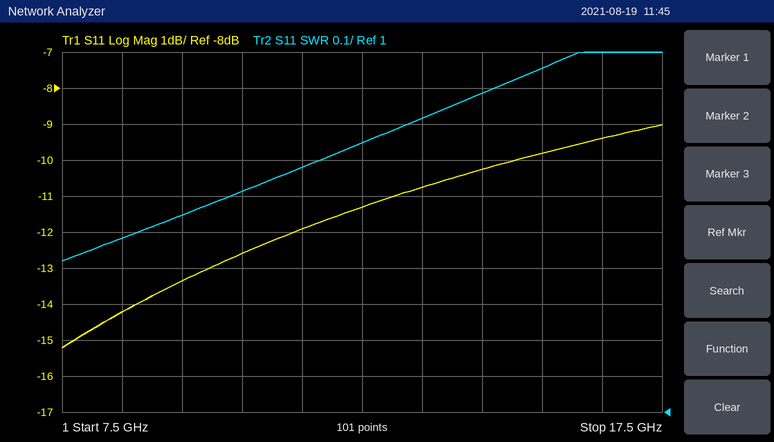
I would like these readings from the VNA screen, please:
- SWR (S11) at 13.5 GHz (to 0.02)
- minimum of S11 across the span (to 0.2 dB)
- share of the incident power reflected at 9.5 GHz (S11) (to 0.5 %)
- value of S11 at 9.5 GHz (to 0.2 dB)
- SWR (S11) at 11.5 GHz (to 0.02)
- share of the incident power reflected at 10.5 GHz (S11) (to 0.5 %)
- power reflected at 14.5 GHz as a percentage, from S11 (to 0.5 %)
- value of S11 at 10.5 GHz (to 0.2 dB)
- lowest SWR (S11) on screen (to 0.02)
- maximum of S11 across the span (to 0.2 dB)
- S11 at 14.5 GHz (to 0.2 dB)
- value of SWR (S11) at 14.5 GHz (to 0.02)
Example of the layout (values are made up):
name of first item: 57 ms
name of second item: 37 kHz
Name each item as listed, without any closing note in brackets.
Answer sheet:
SWR (S11) at 13.5 GHz: 1.82
minimum of S11 across the span: -15.2 dB
share of the incident power reflected at 9.5 GHz (S11): 4.5 %
value of S11 at 9.5 GHz: -13.4 dB
SWR (S11) at 11.5 GHz: 1.68
share of the incident power reflected at 10.5 GHz (S11): 5.5 %
power reflected at 14.5 GHz as a percentage, from S11: 9.5 %
value of S11 at 10.5 GHz: -12.6 dB
lowest SWR (S11) on screen: 1.42
maximum of S11 across the span: -9.0 dB
S11 at 14.5 GHz: -10.2 dB
value of SWR (S11) at 14.5 GHz: 1.88
